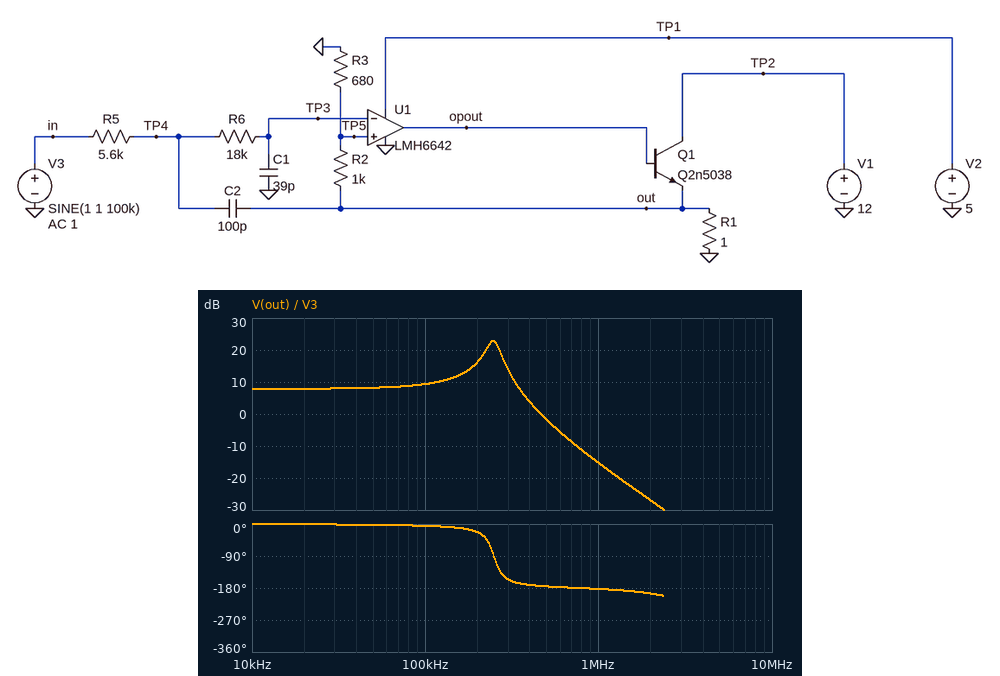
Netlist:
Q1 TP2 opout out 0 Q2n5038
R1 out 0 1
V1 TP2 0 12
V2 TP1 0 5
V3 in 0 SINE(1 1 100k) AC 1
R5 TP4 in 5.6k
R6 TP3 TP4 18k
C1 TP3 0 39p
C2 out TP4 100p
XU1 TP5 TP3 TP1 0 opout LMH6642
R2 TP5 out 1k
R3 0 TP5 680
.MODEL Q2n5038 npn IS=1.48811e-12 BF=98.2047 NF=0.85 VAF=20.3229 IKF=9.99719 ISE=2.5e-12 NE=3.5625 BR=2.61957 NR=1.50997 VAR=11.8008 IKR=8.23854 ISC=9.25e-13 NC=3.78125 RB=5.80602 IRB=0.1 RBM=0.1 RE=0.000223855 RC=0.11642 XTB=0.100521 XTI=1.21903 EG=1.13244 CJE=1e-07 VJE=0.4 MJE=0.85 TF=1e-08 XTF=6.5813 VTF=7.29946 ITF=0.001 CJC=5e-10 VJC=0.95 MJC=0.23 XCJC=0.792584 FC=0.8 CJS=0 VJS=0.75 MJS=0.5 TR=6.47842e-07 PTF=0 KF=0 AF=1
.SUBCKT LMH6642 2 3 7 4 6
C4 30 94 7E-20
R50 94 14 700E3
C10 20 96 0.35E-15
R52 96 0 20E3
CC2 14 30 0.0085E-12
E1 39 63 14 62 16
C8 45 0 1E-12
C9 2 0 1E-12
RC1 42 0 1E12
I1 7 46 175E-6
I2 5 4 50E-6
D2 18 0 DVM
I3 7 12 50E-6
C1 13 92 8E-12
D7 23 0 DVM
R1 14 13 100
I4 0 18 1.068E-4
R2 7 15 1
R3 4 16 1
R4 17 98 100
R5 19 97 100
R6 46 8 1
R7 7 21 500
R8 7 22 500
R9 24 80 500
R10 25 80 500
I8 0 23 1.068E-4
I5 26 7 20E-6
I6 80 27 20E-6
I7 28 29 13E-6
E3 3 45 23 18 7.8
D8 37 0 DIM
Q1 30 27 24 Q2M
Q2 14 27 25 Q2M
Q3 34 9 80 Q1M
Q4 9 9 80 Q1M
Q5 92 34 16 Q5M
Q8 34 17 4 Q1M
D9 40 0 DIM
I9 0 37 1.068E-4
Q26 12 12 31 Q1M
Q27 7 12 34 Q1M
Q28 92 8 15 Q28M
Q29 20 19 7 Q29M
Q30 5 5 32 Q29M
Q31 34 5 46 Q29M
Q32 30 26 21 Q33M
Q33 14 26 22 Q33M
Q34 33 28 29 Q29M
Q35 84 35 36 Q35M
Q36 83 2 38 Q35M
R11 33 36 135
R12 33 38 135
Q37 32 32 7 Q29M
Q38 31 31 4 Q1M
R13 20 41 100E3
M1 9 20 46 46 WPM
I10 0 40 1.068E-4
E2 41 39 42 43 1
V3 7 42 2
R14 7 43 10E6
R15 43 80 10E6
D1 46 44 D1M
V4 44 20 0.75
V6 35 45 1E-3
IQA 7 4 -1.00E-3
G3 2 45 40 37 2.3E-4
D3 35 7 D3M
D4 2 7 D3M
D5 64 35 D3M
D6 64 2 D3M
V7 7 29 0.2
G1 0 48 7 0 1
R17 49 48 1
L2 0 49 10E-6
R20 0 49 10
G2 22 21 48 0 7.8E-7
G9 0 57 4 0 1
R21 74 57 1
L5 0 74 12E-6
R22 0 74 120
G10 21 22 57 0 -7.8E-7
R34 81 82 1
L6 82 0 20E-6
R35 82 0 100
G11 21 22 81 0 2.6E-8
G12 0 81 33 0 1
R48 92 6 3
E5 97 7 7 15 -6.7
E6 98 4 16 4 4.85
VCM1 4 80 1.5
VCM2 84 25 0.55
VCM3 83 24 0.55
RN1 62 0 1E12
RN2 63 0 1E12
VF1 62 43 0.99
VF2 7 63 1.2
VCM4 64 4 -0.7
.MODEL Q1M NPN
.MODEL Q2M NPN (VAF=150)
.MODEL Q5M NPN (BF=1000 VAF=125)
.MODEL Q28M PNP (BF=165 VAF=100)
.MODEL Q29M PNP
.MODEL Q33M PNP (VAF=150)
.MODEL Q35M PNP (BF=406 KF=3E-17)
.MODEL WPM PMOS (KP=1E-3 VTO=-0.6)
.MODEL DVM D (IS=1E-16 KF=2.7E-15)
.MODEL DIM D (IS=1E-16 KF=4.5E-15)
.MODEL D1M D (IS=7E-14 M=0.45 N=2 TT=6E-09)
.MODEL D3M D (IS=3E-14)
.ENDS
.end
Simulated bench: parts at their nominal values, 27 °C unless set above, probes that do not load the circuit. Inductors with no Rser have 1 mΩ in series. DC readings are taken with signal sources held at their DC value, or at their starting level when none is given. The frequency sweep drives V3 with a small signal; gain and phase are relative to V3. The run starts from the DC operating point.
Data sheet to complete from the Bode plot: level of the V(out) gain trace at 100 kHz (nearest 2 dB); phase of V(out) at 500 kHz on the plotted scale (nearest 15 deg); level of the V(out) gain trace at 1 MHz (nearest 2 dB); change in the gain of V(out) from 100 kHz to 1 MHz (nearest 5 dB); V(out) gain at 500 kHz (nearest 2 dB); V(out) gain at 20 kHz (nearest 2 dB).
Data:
10 dB
-180 deg
-16 dB
-25 dB
-2 dB
8 dB
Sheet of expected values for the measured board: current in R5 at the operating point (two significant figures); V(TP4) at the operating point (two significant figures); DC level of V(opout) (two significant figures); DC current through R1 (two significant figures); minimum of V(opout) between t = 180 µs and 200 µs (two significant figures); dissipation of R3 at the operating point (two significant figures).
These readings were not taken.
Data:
1.6 µA
1.0 V
3.3 V
2.6 A
290 mV
1.6 mW
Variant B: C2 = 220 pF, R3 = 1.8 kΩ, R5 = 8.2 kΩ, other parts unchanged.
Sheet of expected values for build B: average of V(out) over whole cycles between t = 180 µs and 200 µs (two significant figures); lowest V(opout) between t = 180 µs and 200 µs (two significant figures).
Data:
1.5 V
270 mV
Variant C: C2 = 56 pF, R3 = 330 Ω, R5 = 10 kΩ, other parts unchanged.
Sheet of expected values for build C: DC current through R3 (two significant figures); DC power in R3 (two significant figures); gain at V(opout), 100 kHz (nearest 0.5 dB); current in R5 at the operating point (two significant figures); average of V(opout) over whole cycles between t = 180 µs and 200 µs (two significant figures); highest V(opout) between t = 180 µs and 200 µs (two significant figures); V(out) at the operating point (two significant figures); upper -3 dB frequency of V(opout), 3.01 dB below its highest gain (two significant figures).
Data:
3.0 mA
2.9 mW
-49.5 dB
1.2 µA
3.0 V
4.7 V
4.0 V
110 kHz
